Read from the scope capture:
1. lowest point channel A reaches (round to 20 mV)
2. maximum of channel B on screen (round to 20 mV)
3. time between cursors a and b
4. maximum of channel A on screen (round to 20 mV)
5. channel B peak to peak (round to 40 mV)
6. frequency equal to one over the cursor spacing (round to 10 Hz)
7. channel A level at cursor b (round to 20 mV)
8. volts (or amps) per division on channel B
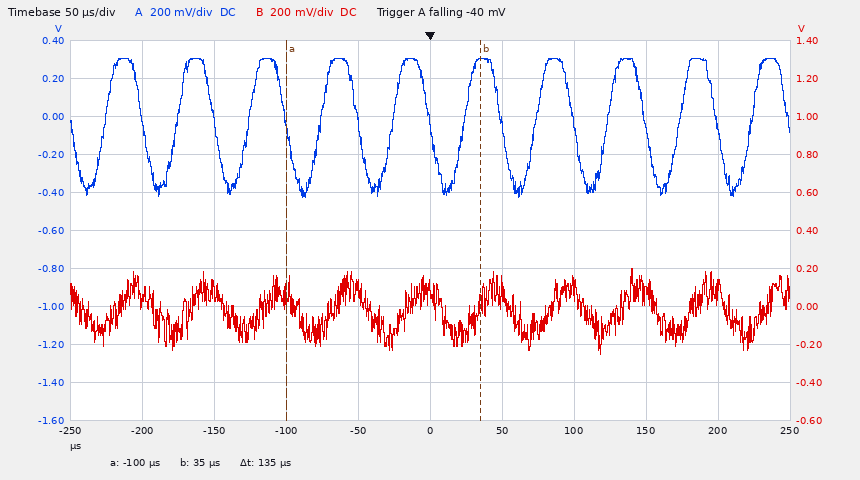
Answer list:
-420 mV
200 mV
135 µs
300 mV
440 mV
7.41 kHz
300 mV
200 mV
